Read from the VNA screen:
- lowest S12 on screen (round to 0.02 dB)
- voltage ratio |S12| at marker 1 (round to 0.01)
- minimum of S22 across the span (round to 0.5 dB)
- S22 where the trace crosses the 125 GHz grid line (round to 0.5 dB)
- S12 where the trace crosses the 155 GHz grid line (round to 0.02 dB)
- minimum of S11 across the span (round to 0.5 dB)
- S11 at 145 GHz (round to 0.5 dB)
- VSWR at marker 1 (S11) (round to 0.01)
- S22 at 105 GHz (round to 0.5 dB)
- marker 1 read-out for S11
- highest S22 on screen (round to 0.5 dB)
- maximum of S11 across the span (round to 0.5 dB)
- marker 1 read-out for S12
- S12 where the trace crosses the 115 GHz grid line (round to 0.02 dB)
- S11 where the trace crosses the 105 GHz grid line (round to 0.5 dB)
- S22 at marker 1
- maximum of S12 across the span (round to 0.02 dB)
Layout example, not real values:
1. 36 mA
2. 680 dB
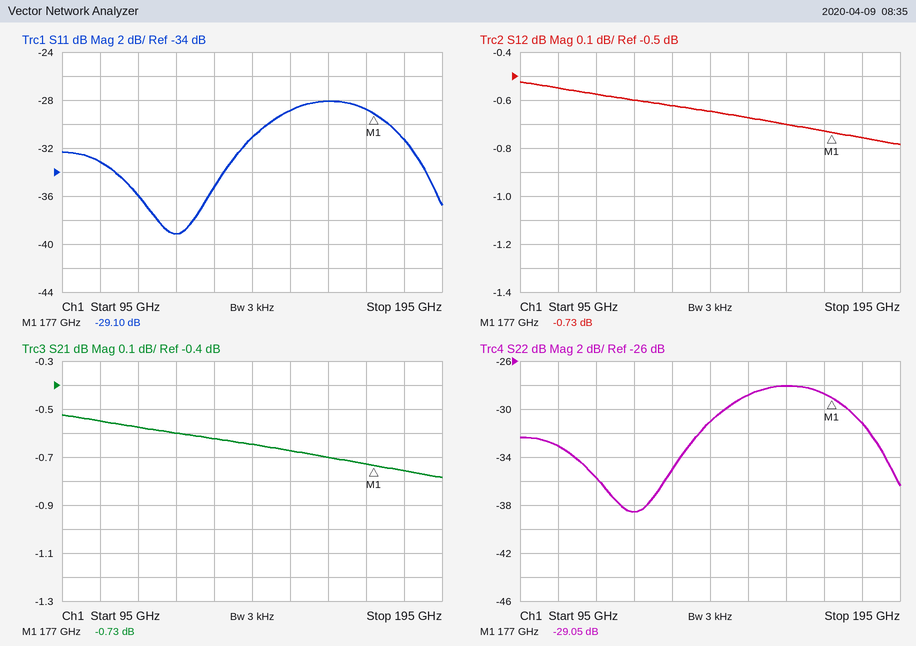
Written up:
1. -0.78 dB
2. 0.92
3. -38.5 dB
4. -38.5 dB
5. -0.68 dB
6. -39.0 dB
7. -31.0 dB
8. 1.07
9. -33.0 dB
10. -29.10 dB
11. -28.0 dB
12. -28.0 dB
13. -0.73 dB
14. -0.58 dB
15. -33.0 dB
16. -29.05 dB
17. -0.52 dB
